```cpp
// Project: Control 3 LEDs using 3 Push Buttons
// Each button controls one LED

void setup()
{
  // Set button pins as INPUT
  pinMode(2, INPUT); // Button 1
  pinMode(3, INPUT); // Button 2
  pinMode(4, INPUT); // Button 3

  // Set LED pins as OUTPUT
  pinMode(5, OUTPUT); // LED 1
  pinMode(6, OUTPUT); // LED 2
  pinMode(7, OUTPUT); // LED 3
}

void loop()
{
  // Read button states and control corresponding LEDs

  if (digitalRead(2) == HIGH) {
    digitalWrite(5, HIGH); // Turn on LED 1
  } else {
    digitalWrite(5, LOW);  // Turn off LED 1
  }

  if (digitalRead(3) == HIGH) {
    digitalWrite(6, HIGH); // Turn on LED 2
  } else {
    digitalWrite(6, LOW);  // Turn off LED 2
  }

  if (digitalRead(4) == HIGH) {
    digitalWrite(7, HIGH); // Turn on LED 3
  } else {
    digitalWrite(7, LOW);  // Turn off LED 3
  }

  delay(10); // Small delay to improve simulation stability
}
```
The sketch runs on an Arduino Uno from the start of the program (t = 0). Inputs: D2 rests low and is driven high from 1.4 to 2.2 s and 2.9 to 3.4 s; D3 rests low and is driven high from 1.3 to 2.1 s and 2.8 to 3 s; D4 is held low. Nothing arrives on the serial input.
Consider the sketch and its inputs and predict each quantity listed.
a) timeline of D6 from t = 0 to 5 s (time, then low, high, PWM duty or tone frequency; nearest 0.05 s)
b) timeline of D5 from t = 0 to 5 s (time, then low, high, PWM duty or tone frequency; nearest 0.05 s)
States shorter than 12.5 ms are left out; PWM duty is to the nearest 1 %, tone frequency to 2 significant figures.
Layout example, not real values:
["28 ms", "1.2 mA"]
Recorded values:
["0 s low; 1.3 s high; 2.1 s low; 2.8 s high; 3 s low", "0 s low; 1.4 s high; 2.2 s low; 2.9 s high; 3.4 s low"]
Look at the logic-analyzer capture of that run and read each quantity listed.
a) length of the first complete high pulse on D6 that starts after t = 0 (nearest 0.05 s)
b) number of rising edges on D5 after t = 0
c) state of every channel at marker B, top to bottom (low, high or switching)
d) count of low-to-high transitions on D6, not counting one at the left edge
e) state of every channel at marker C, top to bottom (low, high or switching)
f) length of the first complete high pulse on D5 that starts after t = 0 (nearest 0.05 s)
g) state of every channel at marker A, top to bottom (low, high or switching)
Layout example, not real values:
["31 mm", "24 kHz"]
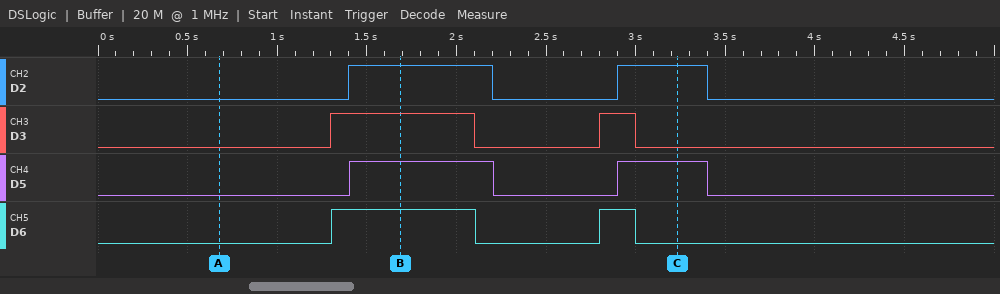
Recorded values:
["0.80 s", "2", "D2 high, D3 high, D5 high, D6 high", "2", "D2 high, D3 low, D5 high, D6 low", "0.80 s", "D2 low, D3 low, D5 low, D6 low"]
